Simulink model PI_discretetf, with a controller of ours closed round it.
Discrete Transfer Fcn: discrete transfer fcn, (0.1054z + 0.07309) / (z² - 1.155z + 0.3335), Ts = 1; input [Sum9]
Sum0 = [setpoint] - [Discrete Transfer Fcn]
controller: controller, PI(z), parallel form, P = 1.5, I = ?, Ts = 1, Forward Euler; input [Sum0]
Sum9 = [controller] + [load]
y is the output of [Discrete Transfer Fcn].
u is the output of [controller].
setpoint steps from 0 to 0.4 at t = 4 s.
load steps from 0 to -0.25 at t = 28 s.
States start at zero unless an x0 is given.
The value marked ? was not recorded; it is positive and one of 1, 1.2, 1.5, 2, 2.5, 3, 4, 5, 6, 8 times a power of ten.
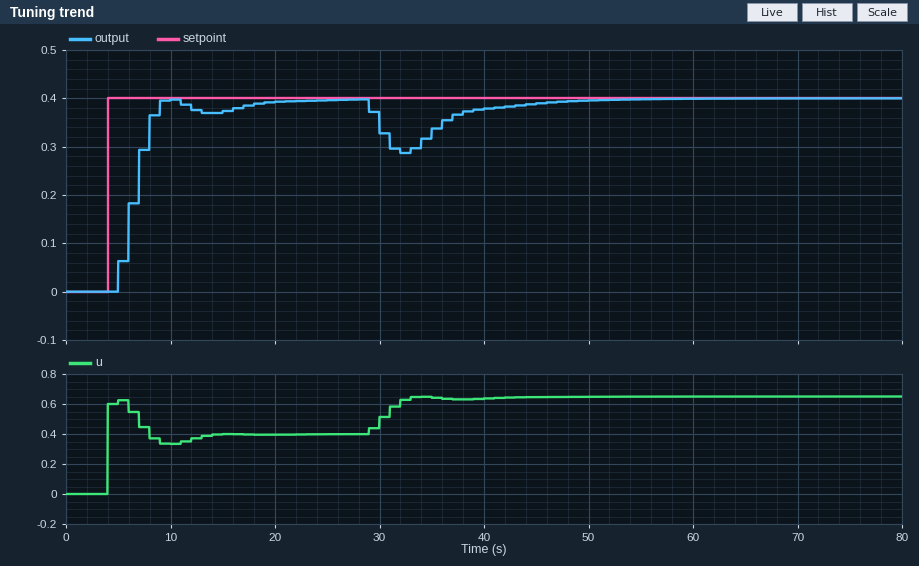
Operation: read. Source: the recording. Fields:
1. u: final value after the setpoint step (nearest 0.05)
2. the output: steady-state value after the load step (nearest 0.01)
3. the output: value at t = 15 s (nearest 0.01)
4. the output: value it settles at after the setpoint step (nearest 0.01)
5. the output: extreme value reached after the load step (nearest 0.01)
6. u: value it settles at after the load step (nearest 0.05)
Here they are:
0.40
0.40
0.37
0.40
0.29
0.65
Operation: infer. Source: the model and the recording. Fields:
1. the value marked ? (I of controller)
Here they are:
0.3
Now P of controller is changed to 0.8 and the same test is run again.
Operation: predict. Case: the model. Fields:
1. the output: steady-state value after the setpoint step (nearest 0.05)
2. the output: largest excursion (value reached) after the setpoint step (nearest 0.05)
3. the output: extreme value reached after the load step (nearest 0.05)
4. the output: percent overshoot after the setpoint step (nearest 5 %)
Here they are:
0.40
0.45
0.25
10 %
